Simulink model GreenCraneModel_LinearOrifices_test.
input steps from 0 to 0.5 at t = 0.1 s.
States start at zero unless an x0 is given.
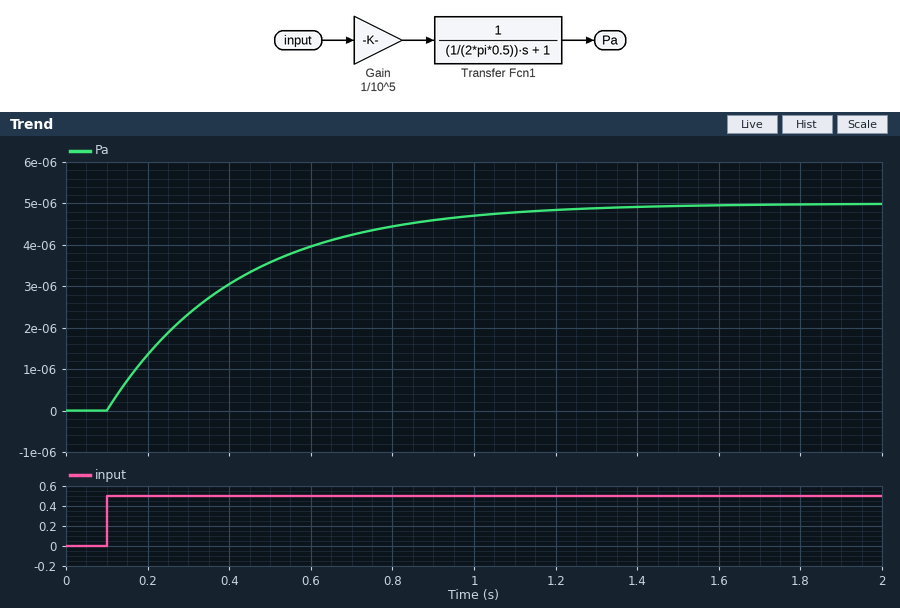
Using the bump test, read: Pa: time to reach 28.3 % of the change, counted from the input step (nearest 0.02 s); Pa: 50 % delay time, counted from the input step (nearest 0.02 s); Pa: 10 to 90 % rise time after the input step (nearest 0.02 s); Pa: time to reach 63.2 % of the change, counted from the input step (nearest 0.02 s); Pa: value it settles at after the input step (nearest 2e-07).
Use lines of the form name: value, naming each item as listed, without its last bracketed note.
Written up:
Pa: time to reach 28.3 % of the change, counted from the input step: 0.10 s
Pa: 50 % delay time, counted from the input step: 0.22 s
Pa: 10 to 90 % rise time after the input step: 0.70 s
Pa: time to reach 63.2 % of the change, counted from the input step: 0.32 s
Pa: value it settles at after the input step: 0.0000050
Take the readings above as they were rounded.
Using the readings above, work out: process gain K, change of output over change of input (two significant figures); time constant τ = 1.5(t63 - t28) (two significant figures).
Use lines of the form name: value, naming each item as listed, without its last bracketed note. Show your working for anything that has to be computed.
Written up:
process gain K, change of output over change of input: (5e-06 - 0) / 0.5 = 0.000010
time constant τ = 1.5(t63 - t28): 1.5 × (0.32 - 0.1) = 0.33 s
